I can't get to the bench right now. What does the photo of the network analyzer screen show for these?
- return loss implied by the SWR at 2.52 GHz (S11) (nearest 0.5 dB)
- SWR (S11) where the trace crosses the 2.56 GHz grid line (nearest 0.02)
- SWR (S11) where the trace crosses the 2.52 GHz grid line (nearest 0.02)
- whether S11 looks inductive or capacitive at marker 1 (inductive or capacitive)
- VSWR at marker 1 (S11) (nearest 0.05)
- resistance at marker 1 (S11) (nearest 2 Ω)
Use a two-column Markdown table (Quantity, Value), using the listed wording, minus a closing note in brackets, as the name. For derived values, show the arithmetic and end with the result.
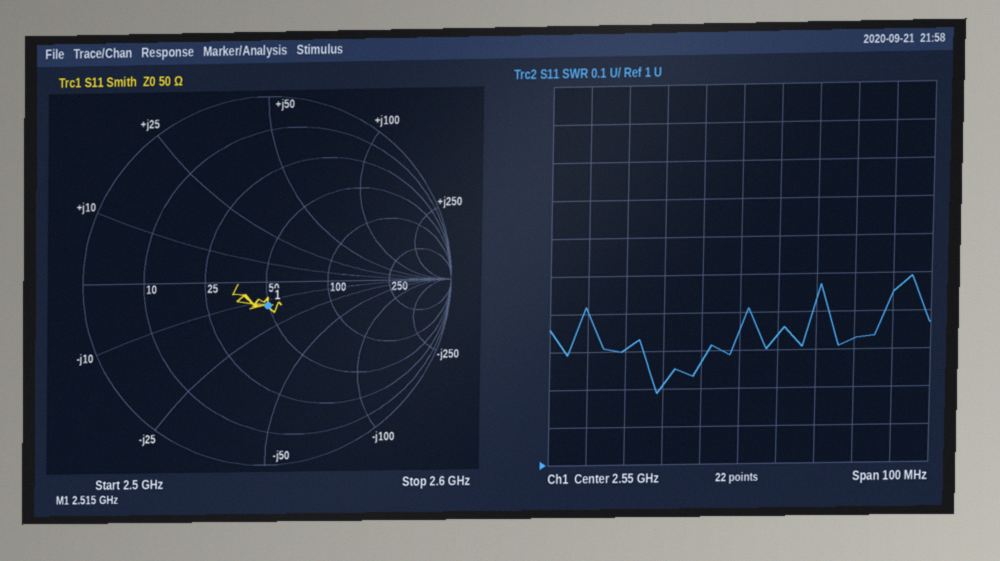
| Quantity | Value |
|---|---|
| return loss implied by the SWR at 2.52 GHz (S11) | −20 log10((1.3 − 1)/(1.3 + 1)) ≈ 17.7 dB, so 17.5 dB to the nearest 0.5 dB |
| SWR (S11) where the trace crosses the 2.56 GHz grid line | 1.34 |
| SWR (S11) where the trace crosses the 2.52 GHz grid line | 1.30 |
| whether S11 looks inductive or capacitive at marker 1 | capacitive |
| VSWR at marker 1 (S11) | 1.30 |
| resistance at marker 1 (S11) | 50 Ω |
